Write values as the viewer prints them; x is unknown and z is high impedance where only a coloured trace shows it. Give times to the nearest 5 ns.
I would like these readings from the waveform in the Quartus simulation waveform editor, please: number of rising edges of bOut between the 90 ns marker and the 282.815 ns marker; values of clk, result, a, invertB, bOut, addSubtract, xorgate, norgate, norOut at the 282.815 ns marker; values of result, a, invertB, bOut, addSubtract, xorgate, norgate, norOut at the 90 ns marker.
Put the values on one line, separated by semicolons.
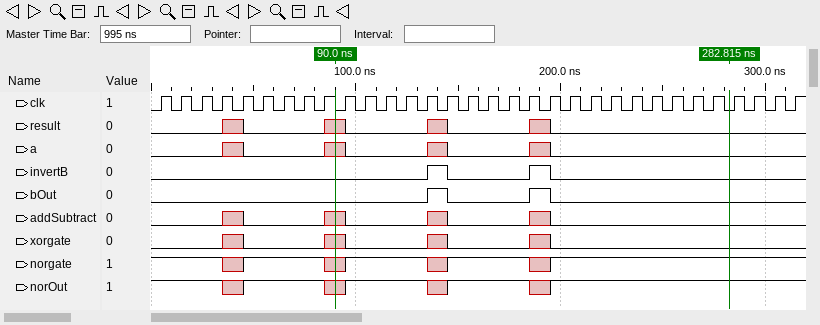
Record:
2; clk=0, result=0, a=0, invertB=0, bOut=0, addSubtract=0, xorgate=0, norgate=1, norOut=1; result=x, a=x, invertB=0, bOut=0, addSubtract=x, xorgate=x, norgate=x, norOut=x
